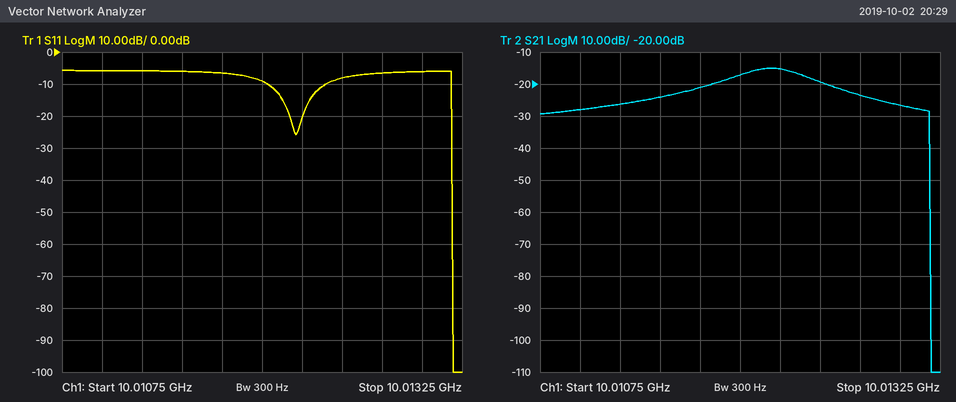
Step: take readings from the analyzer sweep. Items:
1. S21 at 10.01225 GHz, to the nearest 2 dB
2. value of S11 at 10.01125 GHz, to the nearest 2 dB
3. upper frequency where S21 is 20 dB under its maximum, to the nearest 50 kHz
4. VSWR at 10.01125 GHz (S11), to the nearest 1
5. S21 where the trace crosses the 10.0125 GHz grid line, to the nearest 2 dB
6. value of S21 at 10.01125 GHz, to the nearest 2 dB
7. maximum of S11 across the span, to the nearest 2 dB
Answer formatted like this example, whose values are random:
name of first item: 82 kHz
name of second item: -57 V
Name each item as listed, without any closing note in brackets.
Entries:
S21 at 10.01225 GHz, to the nearest 2 dB: -16 dB
value of S11 at 10.01125 GHz, to the nearest 2 dB: -6 dB
upper frequency where S21 is 20 dB under its maximum, to the nearest 50 kHz: 10.01320 GHz
VSWR at 10.01125 GHz (S11), to the nearest 1: 3
S21 where the trace crosses the 10.0125 GHz grid line, to the nearest 2 dB: -20 dB
value of S21 at 10.01125 GHz, to the nearest 2 dB: -26 dB
maximum of S11 across the span, to the nearest 2 dB: -6 dB
